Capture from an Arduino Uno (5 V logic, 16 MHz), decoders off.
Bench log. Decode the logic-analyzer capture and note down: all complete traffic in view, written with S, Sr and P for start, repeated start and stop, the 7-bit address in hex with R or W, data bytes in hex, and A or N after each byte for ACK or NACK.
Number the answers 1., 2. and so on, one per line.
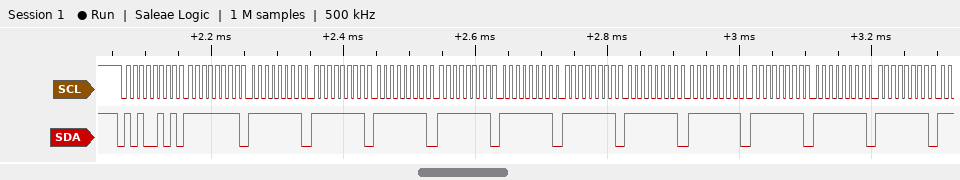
1. S 52R A FF A FF A FF A FF A FF A FF A FF A FF A FF A FF A FF A FF A
